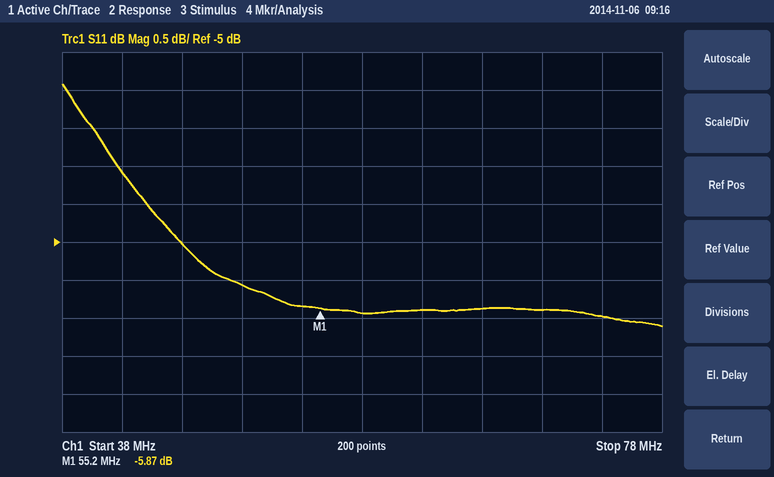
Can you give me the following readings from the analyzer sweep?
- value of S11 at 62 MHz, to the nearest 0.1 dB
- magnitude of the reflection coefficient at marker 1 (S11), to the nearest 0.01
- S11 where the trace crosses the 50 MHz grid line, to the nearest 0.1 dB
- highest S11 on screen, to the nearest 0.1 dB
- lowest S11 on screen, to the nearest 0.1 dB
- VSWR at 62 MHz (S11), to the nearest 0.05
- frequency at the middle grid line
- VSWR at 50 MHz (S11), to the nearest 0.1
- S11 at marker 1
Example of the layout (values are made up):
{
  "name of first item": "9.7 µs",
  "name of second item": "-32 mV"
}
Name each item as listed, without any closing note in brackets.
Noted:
{
  "value of S11 at 62 MHz, to the nearest 0.1 dB": "-5.9 dB",
  "magnitude of the reflection coefficient at marker 1 (S11), to the nearest 0.01": "0.51",
  "S11 where the trace crosses the 50 MHz grid line, to the nearest 0.1 dB": "-5.6 dB",
  "highest S11 on screen, to the nearest 0.1 dB": "-2.9 dB",
  "lowest S11 on screen, to the nearest 0.1 dB": "-6.1 dB",
  "VSWR at 62 MHz (S11), to the nearest 0.05": "3.05",
  "frequency at the middle grid line": "58 MHz",
  "VSWR at 50 MHz (S11), to the nearest 0.1": "3.2",
  "S11 at marker 1": "-5.87 dB"
}
